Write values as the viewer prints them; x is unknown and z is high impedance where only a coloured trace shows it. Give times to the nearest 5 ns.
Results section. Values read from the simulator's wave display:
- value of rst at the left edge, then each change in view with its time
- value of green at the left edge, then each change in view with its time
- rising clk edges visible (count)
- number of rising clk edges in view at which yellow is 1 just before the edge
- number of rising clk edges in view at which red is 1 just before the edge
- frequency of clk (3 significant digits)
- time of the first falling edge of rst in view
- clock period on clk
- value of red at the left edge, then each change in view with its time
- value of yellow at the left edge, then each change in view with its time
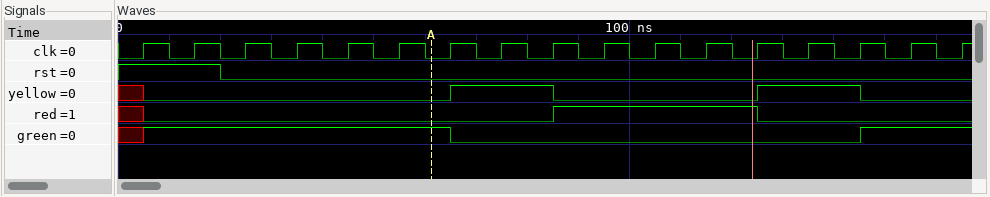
1, 0 at 20 ns
x, 1 at 5 ns, 0 at 65 ns, 1 at 145 ns
17
4
4
100 MHz
20 ns
10 ns
x, 0 at 5 ns, 1 at 85 ns, 0 at 125 ns
x, 0 at 5 ns, 1 at 65 ns, 0 at 85 ns, 1 at 125 ns, 0 at 145 ns
